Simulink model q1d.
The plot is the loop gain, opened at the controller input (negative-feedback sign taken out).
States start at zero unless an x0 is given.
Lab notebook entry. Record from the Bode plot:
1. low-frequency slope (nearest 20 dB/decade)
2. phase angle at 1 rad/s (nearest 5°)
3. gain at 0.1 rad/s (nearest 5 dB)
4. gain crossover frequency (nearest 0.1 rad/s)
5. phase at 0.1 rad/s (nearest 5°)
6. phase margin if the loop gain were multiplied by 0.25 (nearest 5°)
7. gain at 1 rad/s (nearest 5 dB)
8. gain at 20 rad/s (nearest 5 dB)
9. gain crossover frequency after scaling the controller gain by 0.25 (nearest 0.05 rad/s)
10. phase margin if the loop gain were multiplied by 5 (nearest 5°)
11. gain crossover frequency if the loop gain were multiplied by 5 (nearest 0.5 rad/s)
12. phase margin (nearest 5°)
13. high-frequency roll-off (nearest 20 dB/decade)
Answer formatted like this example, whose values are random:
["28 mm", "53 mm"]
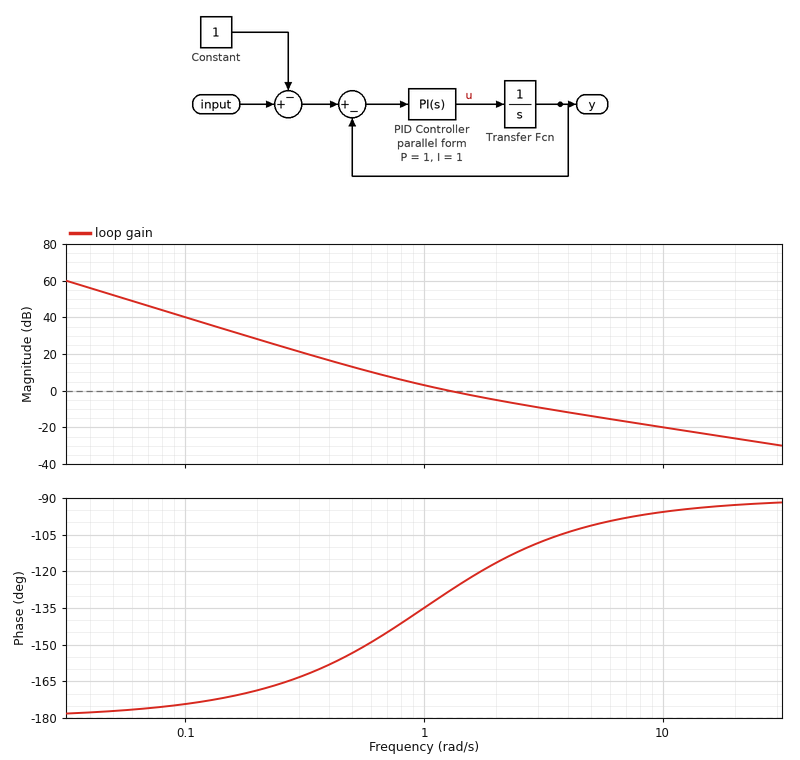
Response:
["-40 dB/decade", "-135°", "40 dB", "1.3 rad/s", "-175°", "30°", "5 dB", "-25 dB", "0.55 rad/s", "80°", "5.0 rad/s", "50°", "-20 dB/decade"]
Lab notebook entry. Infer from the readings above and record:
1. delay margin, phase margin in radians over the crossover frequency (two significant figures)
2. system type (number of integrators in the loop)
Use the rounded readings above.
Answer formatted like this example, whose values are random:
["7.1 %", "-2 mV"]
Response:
["0.67 s", "2"]
